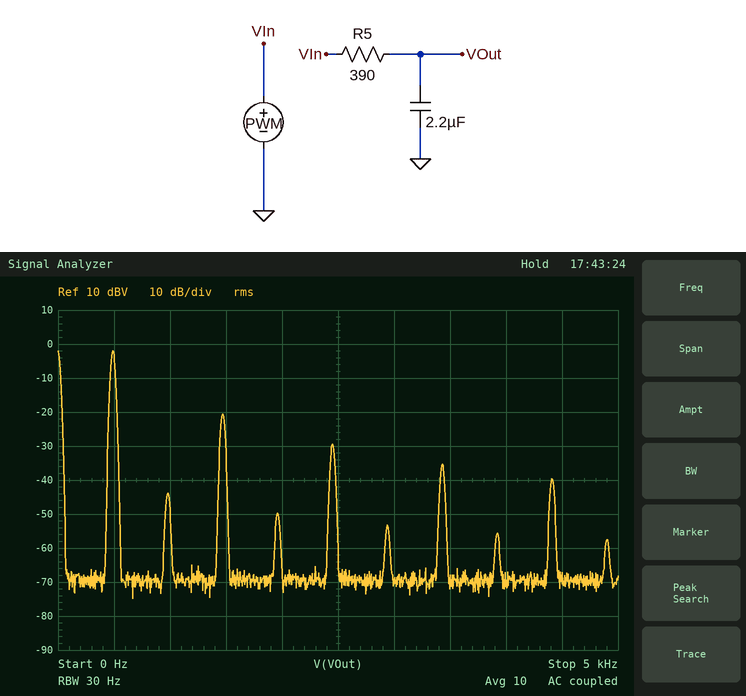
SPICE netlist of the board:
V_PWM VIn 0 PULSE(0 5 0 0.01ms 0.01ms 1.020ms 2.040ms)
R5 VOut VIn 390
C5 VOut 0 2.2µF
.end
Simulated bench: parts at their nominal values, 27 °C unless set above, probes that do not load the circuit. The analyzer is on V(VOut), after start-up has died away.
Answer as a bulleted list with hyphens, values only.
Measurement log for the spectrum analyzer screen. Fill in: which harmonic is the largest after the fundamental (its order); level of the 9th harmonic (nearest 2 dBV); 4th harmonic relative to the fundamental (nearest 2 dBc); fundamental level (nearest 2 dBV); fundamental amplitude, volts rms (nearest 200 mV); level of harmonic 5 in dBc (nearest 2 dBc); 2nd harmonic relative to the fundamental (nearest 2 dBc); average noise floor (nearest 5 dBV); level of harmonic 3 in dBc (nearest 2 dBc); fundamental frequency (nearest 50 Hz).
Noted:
- 3
- -40 dBV
- -48 dBc
- -2 dBV
- 800 mV
- -28 dBc
- -42 dBc
- -70 dBV
- -18 dBc
- 500 Hz
